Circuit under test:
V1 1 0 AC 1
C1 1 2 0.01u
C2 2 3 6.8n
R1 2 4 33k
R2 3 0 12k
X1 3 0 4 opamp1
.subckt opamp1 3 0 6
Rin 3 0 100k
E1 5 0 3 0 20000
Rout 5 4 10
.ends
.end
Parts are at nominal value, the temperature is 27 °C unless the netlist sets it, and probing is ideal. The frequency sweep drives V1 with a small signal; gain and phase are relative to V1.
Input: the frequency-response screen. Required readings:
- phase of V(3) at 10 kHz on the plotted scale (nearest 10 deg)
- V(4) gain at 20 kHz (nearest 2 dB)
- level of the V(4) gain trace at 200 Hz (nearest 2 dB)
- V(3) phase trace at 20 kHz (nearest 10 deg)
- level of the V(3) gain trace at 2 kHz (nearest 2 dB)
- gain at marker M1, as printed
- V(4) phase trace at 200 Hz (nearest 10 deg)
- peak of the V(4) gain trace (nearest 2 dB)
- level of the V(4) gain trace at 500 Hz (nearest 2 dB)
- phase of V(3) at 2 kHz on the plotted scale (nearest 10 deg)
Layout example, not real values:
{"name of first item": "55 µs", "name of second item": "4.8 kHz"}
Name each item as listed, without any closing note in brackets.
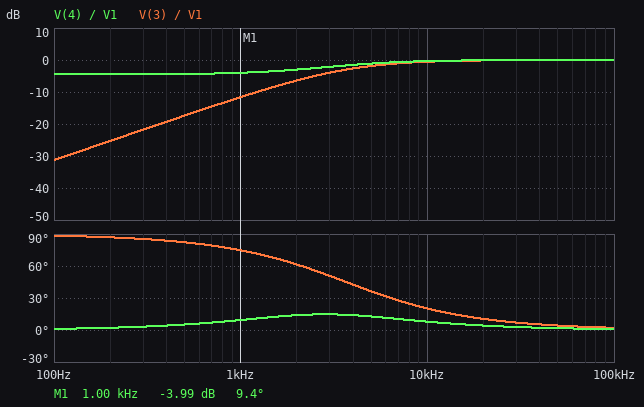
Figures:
{"phase of V(3) at 10 kHz on the plotted scale": "20 deg", "V(4) gain at 20 kHz": "0 dB", "level of the V(4) gain trace at 200 Hz": "-4 dB", "V(3) phase trace at 20 kHz": "10 deg", "level of the V(3) gain trace at 2 kHz": "-6 dB", "gain at marker M1, as printed": "-3.99 dB", "V(4) phase trace at 200 Hz": "0 deg", "peak of the V(4) gain trace": "0 dB", "level of the V(4) gain trace at 500 Hz": "-4 dB", "phase of V(3) at 2 kHz on the plotted scale": "60 deg"}
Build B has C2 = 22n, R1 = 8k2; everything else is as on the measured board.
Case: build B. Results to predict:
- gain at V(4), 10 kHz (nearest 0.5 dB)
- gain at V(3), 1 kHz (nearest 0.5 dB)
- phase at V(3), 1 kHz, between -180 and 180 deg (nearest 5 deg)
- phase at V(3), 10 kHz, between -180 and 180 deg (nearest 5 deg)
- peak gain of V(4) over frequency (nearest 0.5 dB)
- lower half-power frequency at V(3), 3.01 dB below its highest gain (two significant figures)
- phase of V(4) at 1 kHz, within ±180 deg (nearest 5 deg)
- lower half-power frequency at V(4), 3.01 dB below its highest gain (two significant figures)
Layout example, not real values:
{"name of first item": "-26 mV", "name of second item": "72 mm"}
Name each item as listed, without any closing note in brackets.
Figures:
{"gain at V(4), 10 kHz": "0 dB", "gain at V(3), 1 kHz": "-7.5 dB", "phase at V(3), 1 kHz, between -180 and 180 deg": "65 deg", "phase at V(3), 10 kHz, between -180 and 180 deg": "10 deg", "peak gain of V(4) over frequency": "0 dB", "lower half-power frequency at V(3), 3.01 dB below its highest gain": "2.2 kHz", "phase of V(4) at 1 kHz, within ±180 deg": "30 deg", "lower half-power frequency at V(4), 3.01 dB below its highest gain": "1.9 kHz"}
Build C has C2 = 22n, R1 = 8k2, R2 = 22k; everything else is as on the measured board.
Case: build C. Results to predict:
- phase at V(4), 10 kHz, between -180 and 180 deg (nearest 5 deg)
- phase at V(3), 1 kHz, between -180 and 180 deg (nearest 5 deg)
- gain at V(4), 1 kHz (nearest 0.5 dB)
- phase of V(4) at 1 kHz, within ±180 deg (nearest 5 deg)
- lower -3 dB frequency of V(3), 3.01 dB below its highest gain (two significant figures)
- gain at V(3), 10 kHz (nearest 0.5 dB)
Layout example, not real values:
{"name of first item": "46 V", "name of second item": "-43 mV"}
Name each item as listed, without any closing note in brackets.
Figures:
{"phase at V(4), 10 kHz, between -180 and 180 deg": "5 deg", "phase at V(3), 1 kHz, between -180 and 180 deg": "50 deg", "gain at V(4), 1 kHz": "-3.5 dB", "phase of V(4) at 1 kHz, within ±180 deg": "30 deg", "lower -3 dB frequency of V(3), 3.01 dB below its highest gain": "1.3 kHz", "gain at V(3), 10 kHz": "0 dB"}
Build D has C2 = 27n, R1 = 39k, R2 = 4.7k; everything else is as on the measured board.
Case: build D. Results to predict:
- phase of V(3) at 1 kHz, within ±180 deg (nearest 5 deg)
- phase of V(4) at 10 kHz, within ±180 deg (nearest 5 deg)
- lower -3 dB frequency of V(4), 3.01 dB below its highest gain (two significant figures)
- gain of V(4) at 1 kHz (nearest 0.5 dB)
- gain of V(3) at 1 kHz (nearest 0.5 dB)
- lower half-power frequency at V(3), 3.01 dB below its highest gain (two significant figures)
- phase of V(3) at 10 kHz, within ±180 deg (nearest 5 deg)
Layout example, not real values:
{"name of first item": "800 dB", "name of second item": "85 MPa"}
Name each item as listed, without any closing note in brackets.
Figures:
{"phase of V(3) at 1 kHz, within ±180 deg": "80 deg", "phase of V(4) at 10 kHz, within ±180 deg": "20 deg", "lower -3 dB frequency of V(4), 3.01 dB below its highest gain": "4.5 kHz", "gain of V(4) at 1 kHz": "-9.5 dB", "gain of V(3) at 1 kHz": "-14.0 dB", "lower half-power frequency at V(3), 3.01 dB below its highest gain": "4.9 kHz", "phase of V(3) at 10 kHz, within ±180 deg": "25 deg"}
